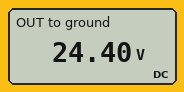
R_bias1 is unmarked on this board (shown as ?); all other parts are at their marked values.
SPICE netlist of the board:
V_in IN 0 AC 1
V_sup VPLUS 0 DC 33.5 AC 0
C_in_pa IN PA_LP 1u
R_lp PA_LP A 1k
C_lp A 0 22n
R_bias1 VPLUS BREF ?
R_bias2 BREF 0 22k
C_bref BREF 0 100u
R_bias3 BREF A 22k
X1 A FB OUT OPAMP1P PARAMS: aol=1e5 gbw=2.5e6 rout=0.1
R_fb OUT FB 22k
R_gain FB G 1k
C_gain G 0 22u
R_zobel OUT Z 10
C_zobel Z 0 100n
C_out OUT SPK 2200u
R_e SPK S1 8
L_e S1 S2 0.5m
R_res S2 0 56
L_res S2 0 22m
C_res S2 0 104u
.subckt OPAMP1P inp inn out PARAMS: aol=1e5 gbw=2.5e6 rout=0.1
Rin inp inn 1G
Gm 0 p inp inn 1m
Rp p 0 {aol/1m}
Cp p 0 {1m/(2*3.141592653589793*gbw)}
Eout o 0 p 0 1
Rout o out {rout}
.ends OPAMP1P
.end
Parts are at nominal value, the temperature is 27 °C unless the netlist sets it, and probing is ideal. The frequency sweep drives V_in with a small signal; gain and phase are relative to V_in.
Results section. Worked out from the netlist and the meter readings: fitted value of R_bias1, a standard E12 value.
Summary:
8.2 kΩ
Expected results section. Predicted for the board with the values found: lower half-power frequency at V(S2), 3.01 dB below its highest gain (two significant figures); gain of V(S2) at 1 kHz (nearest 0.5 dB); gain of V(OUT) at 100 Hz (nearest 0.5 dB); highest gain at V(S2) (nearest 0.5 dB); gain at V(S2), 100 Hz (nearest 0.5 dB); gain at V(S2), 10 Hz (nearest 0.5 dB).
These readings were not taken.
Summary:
39 Hz
12.0 dB
26.5 dB
25.5 dB
25.5 dB
6.0 dB
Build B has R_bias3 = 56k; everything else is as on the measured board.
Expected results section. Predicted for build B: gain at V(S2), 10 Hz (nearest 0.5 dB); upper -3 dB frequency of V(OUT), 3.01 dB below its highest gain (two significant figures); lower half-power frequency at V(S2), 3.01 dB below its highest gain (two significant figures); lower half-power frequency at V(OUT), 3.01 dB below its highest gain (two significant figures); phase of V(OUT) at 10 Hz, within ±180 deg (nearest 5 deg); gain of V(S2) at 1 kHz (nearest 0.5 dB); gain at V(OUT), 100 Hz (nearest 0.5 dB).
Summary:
7.5 dB
7.5 kHz
38 Hz
8.1 Hz
50 deg
12.5 dB
27.0 dB
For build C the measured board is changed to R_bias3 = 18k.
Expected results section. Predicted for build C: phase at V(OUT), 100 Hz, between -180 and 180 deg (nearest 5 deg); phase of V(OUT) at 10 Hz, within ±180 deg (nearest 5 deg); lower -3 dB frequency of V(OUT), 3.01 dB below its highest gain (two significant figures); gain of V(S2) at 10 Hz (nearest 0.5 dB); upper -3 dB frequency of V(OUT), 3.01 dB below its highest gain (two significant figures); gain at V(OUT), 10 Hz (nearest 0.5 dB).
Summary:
10 deg
75 deg
12 Hz
5.5 dB
7.8 kHz
22.5 dB
